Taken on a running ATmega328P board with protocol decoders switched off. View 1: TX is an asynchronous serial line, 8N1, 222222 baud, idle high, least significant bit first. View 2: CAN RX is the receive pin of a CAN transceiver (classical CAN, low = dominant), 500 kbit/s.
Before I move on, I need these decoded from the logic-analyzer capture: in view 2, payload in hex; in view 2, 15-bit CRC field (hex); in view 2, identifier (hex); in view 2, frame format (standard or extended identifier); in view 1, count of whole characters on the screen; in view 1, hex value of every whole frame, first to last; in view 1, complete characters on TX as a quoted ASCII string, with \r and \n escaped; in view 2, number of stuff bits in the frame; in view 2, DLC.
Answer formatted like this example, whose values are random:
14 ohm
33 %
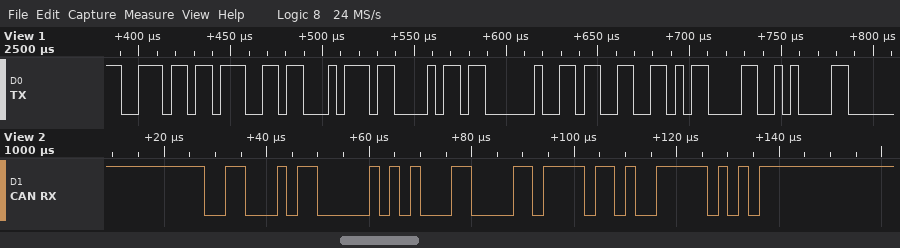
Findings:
8C 37
0x5A7E
0x316
standard
8
6E 67 74 68 20 33 0D 0A
"ngth 3\r\n"
2
2
